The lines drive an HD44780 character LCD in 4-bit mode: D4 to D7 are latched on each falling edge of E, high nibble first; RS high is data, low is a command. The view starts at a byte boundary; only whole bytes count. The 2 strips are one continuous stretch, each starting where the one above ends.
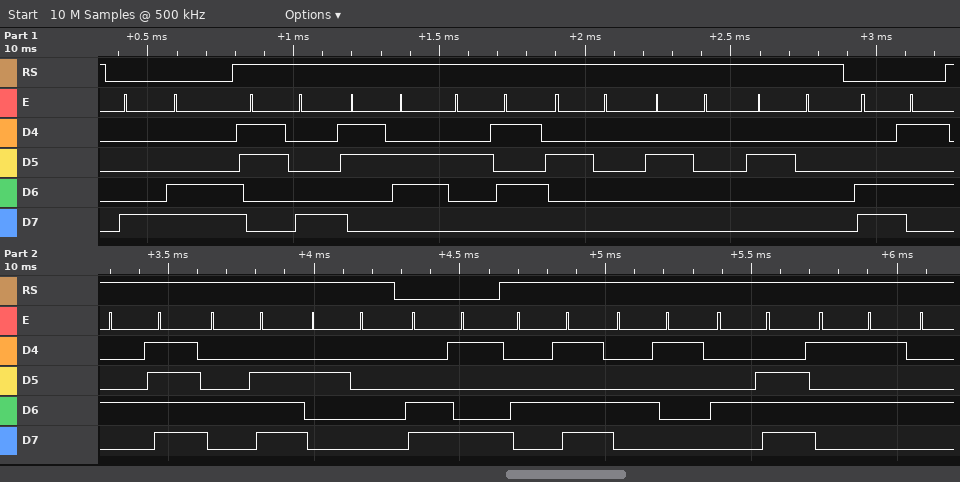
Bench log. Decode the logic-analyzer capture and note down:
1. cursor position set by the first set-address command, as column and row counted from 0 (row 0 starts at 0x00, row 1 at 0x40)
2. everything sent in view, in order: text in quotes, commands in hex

column 12, row 0
0x8C "86%   " 0xC5 "ON " 0xC9 "MANU"
